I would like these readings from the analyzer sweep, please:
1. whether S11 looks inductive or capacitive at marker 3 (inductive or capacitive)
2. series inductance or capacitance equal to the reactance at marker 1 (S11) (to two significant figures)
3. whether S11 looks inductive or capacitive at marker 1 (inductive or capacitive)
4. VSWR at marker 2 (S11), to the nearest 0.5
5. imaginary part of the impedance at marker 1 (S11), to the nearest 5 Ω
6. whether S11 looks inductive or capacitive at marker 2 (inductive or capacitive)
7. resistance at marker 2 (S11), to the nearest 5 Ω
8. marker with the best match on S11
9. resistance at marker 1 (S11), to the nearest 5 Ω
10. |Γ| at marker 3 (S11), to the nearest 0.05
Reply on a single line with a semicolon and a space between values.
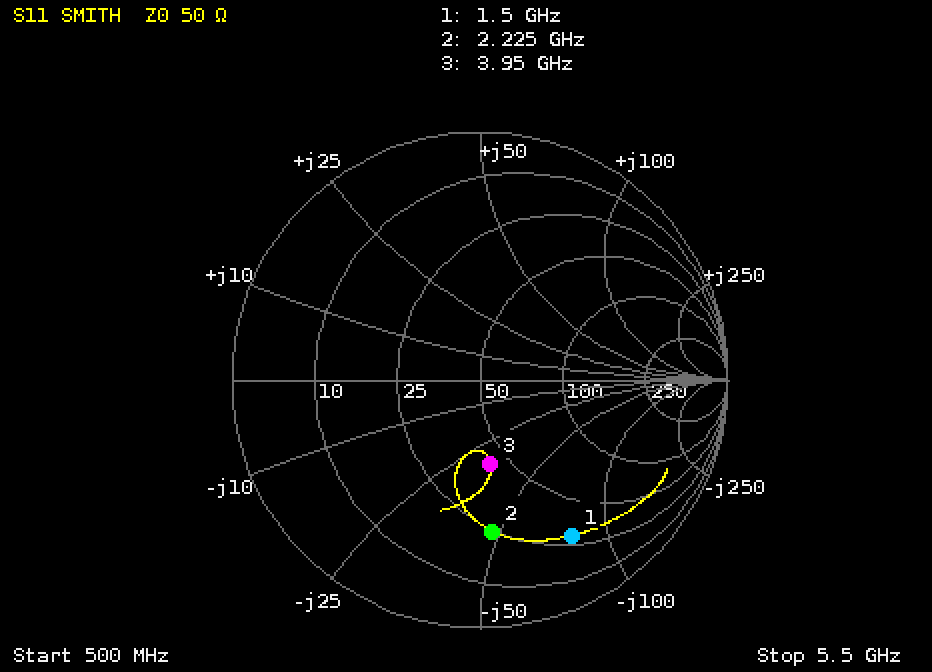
capacitive; 1.3 pF; capacitive; 4.0; -80 Ω; capacitive; 25 Ω; marker 3; 30 Ω; 0.35
